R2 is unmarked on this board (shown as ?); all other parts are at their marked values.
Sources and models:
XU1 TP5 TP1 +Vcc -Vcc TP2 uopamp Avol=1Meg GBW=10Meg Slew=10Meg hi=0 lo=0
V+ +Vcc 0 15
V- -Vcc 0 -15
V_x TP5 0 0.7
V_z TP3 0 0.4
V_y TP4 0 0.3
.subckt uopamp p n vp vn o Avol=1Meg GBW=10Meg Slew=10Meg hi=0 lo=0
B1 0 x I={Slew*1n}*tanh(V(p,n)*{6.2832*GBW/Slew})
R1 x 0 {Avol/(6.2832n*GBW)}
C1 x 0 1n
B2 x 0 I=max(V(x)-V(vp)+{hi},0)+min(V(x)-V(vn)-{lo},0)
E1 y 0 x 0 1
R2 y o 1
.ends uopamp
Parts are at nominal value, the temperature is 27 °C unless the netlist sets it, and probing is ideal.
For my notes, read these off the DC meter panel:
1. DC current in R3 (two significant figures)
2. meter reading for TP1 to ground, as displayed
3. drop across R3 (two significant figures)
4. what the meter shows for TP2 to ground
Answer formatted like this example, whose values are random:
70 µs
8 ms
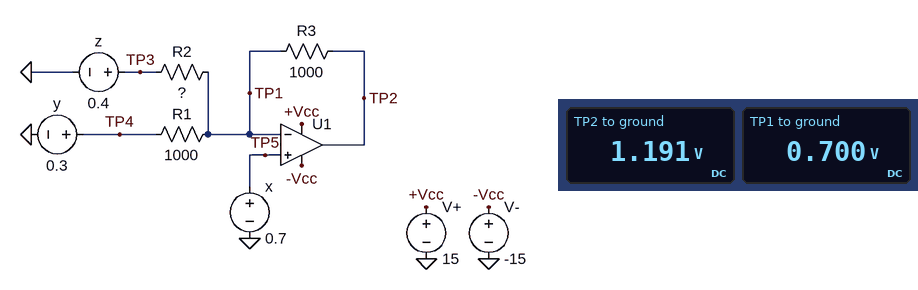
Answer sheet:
490 µA
0.700 V
490 mV
1.191 V
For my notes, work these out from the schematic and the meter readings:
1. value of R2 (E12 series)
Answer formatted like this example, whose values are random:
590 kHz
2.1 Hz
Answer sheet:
3.3 kΩ
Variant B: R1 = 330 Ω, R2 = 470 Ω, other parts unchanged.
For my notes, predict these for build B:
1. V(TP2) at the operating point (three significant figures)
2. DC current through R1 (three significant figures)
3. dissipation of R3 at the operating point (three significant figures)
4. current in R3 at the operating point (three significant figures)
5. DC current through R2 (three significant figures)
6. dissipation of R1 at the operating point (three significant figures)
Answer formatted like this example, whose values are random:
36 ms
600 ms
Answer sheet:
2.55 V
1.21 mA
3.42 mW
1.85 mA
638 µA
485 µW
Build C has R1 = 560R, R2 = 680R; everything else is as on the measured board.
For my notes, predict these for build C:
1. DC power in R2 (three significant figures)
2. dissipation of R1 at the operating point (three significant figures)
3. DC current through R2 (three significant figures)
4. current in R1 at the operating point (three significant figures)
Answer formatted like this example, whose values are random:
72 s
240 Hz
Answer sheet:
132 µW
286 µW
441 µA
714 µA
